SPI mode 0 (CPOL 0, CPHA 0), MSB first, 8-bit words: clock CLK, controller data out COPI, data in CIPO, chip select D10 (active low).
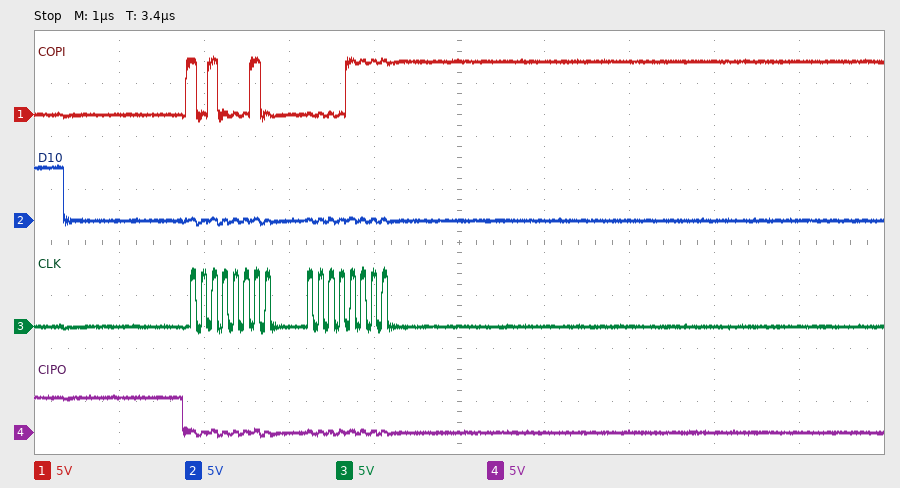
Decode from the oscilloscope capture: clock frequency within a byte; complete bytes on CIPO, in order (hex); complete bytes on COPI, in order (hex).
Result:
8 MHz
00 00
A2 0F
